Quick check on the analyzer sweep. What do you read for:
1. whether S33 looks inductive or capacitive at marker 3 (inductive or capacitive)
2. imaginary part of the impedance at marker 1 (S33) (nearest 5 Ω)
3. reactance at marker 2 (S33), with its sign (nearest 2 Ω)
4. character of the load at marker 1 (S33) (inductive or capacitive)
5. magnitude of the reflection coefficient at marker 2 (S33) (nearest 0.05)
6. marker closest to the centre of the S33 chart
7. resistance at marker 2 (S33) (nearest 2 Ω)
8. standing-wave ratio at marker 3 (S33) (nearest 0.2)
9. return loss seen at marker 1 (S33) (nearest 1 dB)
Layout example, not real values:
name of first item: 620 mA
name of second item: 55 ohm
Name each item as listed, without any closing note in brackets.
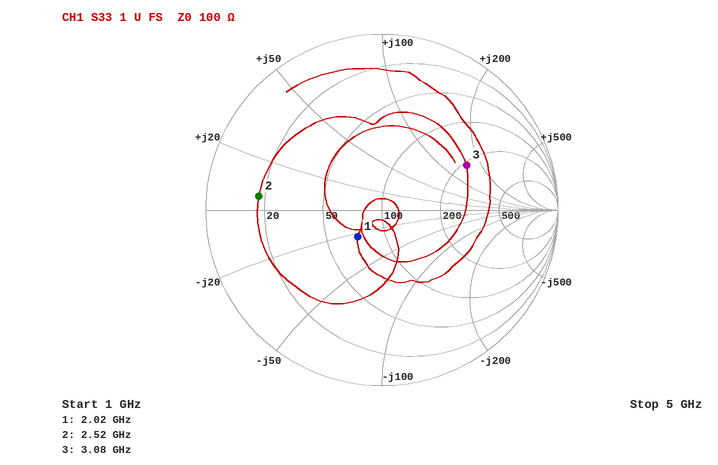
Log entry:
whether S33 looks inductive or capacitive at marker 3: inductive
imaginary part of the impedance at marker 1 (S33): -25 Ω
reactance at marker 2 (S33), with its sign: +6 Ω
character of the load at marker 1 (S33): capacitive
magnitude of the reflection coefficient at marker 2 (S33): 0.70
marker closest to the centre of the S33 chart: marker 1
resistance at marker 2 (S33): 18 Ω
standing-wave ratio at marker 3 (S33): 3.4
return loss seen at marker 1 (S33): 14 dB
